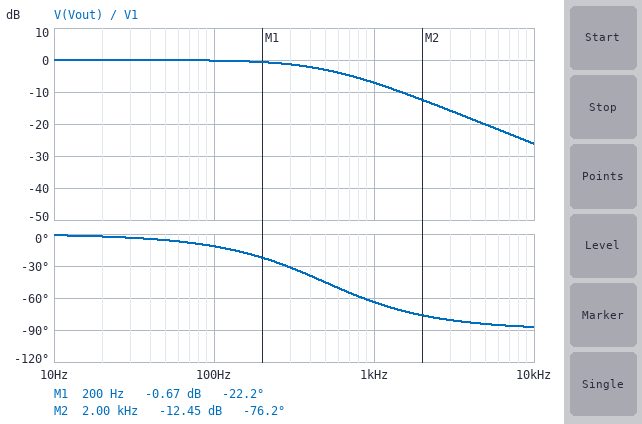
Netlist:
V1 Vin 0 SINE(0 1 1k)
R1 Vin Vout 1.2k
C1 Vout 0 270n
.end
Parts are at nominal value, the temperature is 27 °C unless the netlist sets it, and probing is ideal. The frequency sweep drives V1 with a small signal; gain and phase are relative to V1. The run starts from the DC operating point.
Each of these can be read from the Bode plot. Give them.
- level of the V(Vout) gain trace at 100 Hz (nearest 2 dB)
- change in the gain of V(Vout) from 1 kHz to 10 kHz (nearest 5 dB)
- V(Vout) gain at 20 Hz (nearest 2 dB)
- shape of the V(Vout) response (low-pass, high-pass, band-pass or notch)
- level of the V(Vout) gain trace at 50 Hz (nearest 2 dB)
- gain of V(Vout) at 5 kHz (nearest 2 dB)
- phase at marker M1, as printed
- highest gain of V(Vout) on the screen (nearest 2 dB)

0 dB
-20 dB
0 dB
low-pass
0 dB
-20 dB
-22.2 deg
0 dB
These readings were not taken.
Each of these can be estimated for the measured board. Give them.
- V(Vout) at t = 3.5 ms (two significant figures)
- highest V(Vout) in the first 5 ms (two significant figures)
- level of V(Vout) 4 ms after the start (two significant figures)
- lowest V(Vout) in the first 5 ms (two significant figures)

400 mV
550 mV
-400 mV
-440 mV
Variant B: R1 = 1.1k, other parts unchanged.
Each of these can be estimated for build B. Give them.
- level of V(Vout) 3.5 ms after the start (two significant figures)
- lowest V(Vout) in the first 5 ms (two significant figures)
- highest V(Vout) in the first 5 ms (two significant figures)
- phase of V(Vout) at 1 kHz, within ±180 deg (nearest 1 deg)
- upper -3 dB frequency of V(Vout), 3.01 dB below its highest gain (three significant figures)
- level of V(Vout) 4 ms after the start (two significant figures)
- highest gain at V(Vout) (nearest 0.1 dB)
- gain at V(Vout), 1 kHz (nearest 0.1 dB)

420 mV
-470 mV
580 mV
-62 deg
536 Hz
-420 mV
0 dB
-6.5 dB
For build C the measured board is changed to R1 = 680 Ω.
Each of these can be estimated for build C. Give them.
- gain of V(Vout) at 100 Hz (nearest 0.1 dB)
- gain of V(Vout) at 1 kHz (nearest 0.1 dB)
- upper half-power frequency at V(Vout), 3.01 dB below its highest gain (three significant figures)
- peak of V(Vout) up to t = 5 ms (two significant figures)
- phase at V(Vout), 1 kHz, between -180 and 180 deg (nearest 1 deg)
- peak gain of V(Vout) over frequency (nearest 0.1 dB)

-0.1 dB
-3.7 dB
867 Hz
720 mV
-49 deg
0 dB
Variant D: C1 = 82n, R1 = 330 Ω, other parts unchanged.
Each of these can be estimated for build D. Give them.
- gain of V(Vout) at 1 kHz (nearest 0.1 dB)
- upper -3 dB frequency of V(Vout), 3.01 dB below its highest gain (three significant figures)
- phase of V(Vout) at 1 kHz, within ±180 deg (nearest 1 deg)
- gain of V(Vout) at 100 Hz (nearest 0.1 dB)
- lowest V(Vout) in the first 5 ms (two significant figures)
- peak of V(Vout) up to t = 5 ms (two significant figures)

-0.1 dB
5.88 kHz
-10 deg
0 dB
-990 mV
990 mV
